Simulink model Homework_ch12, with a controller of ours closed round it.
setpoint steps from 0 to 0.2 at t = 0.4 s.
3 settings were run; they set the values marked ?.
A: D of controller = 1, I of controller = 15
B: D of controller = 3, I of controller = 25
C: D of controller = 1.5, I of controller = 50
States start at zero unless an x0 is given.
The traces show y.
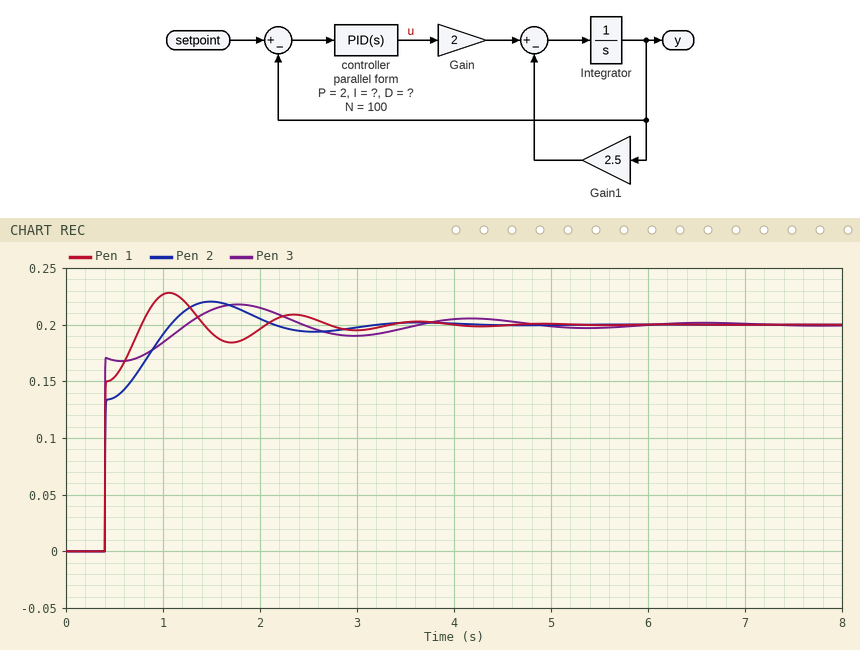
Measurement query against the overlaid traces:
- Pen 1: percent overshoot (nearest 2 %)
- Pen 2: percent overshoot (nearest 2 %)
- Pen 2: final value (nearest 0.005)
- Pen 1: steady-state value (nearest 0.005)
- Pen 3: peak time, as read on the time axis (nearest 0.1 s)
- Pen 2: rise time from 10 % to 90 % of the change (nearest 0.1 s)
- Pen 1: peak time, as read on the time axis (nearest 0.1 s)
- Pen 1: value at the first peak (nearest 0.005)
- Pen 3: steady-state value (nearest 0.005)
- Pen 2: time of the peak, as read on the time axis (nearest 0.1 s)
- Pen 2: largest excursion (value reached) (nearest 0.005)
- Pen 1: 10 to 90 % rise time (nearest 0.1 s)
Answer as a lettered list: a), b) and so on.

a) 14 %
b) 10 %
c) 0.200
d) 0.200
e) 1.8 s
f) 0.5 s
g) 1.1 s
h) 0.230
i) 0.200
j) 1.5 s
k) 0.220
l) 0.3 s
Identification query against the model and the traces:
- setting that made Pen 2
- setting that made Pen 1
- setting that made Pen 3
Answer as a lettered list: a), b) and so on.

a) A
b) C
c) B
